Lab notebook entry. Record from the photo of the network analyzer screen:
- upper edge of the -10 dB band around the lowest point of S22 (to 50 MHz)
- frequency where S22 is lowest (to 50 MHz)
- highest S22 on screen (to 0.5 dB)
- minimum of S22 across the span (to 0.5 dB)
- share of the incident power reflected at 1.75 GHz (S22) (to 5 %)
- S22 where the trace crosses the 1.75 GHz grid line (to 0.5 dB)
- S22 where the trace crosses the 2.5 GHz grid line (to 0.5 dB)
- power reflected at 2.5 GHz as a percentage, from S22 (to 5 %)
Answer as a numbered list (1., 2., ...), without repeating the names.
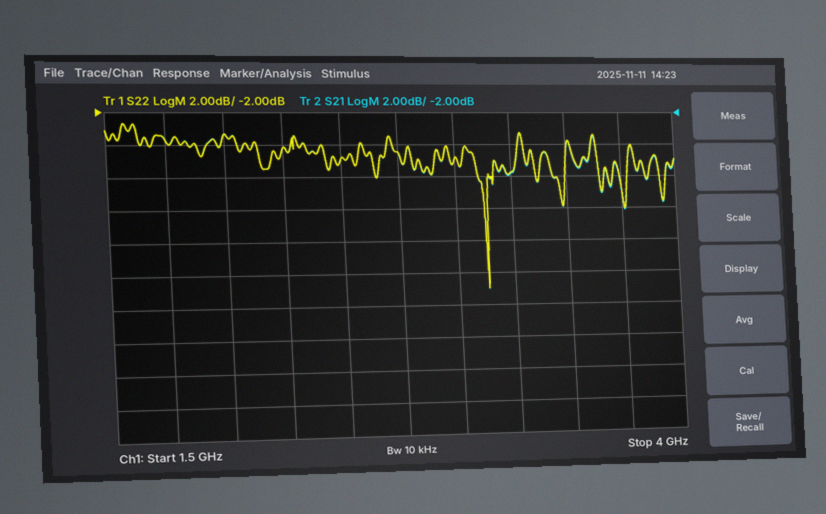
1. 3.15 GHz
2. 3.15 GHz
3. -2.5 dB
4. -13.0 dB
5. 45 %
6. -3.5 dB
7. -5.0 dB
8. 30 %
